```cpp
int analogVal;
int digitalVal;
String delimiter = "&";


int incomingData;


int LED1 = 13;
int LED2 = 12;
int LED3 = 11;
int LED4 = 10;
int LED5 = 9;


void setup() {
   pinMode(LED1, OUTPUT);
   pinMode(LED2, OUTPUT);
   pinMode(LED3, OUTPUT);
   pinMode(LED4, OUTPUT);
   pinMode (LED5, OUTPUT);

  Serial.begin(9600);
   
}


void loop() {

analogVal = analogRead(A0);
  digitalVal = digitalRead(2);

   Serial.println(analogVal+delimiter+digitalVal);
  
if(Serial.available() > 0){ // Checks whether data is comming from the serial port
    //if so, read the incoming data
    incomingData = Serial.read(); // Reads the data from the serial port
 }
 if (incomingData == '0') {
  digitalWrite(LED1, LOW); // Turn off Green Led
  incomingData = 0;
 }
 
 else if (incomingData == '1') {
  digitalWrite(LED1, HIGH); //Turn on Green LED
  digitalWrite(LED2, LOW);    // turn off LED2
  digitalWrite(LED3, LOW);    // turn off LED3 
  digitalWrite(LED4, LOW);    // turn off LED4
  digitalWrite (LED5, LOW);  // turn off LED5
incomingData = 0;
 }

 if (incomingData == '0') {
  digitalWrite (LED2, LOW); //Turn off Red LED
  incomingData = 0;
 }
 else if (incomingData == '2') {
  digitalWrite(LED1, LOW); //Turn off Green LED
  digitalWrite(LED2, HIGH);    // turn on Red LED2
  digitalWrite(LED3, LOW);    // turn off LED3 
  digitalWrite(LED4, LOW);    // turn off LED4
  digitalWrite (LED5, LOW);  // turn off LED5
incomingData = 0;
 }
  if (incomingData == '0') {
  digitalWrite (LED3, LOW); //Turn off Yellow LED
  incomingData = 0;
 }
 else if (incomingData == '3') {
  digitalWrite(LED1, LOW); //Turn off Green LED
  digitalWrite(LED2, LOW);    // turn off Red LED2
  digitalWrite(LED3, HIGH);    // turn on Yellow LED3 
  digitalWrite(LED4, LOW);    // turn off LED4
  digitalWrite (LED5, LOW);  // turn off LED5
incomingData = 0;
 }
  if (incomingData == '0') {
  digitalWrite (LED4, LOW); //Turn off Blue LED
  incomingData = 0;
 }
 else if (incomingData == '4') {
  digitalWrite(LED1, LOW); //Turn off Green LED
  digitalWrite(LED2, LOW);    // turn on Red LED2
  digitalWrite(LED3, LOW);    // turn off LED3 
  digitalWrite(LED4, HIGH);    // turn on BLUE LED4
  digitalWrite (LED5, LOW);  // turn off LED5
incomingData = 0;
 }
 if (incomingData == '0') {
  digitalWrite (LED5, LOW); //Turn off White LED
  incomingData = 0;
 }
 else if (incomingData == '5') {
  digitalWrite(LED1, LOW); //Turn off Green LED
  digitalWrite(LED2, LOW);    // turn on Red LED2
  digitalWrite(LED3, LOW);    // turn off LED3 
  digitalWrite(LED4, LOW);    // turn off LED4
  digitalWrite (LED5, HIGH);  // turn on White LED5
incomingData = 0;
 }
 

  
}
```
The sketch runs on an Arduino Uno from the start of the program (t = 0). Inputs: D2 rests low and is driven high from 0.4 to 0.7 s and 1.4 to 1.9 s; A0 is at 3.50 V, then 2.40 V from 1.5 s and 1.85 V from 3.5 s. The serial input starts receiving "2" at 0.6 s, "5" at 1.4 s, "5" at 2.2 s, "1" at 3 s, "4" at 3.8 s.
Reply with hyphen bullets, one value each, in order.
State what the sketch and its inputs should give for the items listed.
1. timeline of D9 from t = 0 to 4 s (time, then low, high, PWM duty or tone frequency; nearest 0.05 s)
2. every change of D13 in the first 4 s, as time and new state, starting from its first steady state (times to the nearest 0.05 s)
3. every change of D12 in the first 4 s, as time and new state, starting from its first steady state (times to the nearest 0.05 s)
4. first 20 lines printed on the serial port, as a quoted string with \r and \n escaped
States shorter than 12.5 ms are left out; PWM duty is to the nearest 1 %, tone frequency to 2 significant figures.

- 0 s low; 1.4 s high; 3 s low
- 0 s low; 3 s high; 3.8 s low
- 0 s low; 0.6 s high; 1.4 s low
- "716&0\r\n716&0\r\n716&0\r\n716&0\r\n716&0\r\n716&0\r\n716&0\r\n716&0\r\n716&0\r\n716&0\r\n716&0\r\n716&0\r\n716&0\r\n716&0\r\n716&0\r\n716&0\r\n716&0\r\n716&0\r\n716&0\r\n716&0\r\n"
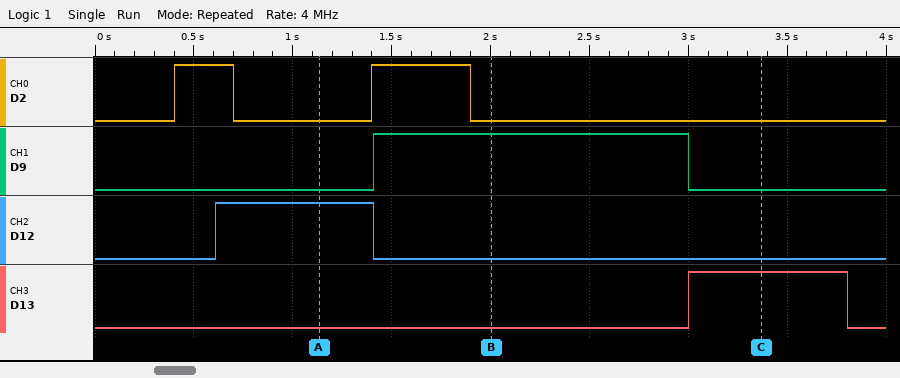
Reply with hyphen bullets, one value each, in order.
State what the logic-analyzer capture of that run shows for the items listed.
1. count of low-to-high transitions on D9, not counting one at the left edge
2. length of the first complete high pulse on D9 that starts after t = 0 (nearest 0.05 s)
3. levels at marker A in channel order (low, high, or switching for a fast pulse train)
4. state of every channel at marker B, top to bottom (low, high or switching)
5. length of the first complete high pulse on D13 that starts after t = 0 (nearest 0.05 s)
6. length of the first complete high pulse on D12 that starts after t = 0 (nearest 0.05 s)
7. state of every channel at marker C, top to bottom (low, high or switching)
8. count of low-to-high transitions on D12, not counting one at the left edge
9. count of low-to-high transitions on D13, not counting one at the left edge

- 1
- 1.60 s
- D2 low, D9 low, D12 high, D13 low
- D2 low, D9 high, D12 low, D13 low
- 0.80 s
- 0.80 s
- D2 low, D9 low, D12 low, D13 high
- 1
- 1
